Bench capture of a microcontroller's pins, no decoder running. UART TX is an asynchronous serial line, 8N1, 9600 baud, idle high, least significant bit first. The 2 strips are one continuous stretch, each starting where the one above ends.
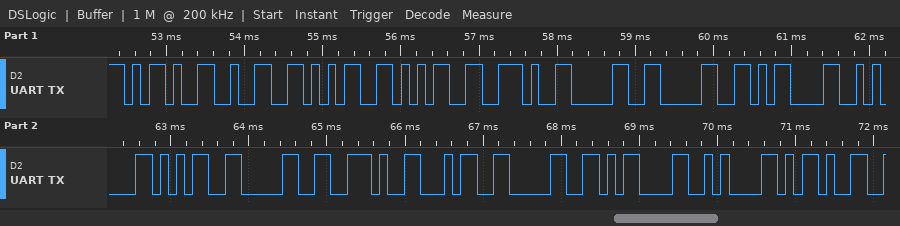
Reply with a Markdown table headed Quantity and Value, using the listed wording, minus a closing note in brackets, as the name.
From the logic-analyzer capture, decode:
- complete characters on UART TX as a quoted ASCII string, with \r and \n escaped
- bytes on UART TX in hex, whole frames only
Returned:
| Quantity | Value |
|---|---|
| complete characters on UART TX as a quoted ASCII string, with \r and \n escaped | "-255.00\r\n50.40\r\n-" |
| bytes on UART TX in hex, whole frames only | 2D 32 35 35 2E 30 30 0D 0A 35 30 2E 34 30 0D 0A 2D |
